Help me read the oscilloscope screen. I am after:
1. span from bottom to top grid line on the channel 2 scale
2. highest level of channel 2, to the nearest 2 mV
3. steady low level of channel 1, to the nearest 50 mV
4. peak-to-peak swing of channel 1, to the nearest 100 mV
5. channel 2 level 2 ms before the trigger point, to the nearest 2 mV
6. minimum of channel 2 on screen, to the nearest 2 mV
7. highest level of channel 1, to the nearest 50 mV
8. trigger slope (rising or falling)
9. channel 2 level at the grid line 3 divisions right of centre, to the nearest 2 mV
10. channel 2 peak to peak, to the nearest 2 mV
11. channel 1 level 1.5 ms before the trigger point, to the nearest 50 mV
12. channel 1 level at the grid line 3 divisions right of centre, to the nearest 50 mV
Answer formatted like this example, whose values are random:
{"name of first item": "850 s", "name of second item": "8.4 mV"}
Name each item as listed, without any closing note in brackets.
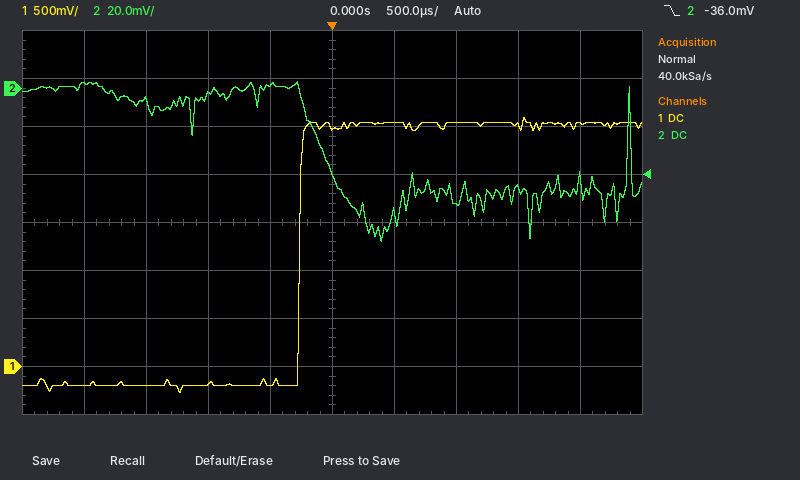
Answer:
{"span from bottom to top grid line on the channel 2 scale": "160 mV", "highest level of channel 2, to the nearest 2 mV": "2 mV", "steady low level of channel 1, to the nearest 50 mV": "-200 mV", "peak-to-peak swing of channel 1, to the nearest 100 mV": "2.90 V", "channel 2 level 2 ms before the trigger point, to the nearest 2 mV": "2 mV", "minimum of channel 2 on screen, to the nearest 2 mV": "-64 mV", "highest level of channel 1, to the nearest 50 mV": "2.60 V", "trigger slope": "falling", "channel 2 level at the grid line 3 divisions right of centre, to the nearest 2 mV": "-42 mV", "channel 2 peak to peak, to the nearest 2 mV": "66 mV", "channel 1 level 1.5 ms before the trigger point, to the nearest 50 mV": "-200 mV", "channel 1 level at the grid line 3 divisions right of centre, to the nearest 50 mV": "2.50 V"}
